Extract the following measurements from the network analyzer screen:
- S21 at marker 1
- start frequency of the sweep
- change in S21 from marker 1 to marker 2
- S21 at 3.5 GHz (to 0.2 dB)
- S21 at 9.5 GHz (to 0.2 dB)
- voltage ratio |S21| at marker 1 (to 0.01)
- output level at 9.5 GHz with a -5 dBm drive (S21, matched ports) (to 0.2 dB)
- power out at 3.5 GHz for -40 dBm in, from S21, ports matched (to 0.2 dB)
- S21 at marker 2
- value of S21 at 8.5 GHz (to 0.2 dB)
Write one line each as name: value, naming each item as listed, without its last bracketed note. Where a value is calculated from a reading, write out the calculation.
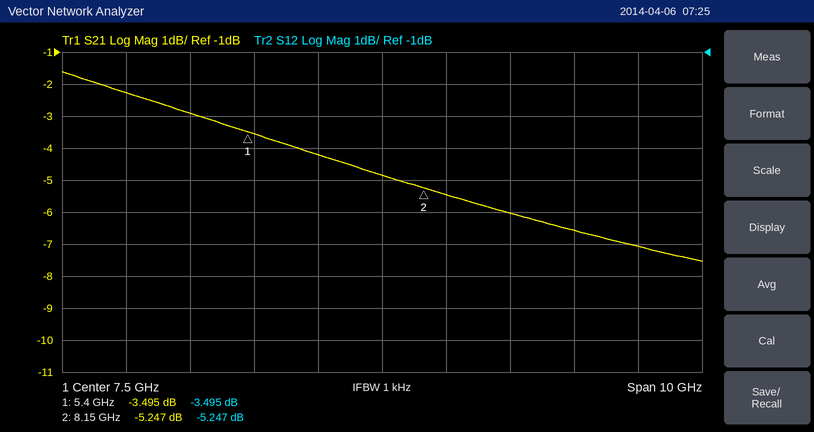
S21 at marker 1: -3.495 dB
start frequency of the sweep: 2.5 GHz
change in S21 from marker 1 to marker 2: -5.247 − (-3.495) = -1.752 dB
S21 at 3.5 GHz: -2.2 dB
S21 at 9.5 GHz: -6.0 dB
voltage ratio |S21| at marker 1: 10^(-3.495/20) ≈ 0.67
output level at 9.5 GHz with a -5 dBm drive (S21, matched ports): -5 dBm + (-6.0 dB) = -11.0 dBm
power out at 3.5 GHz for -40 dBm in, from S21, ports matched: -40 dBm + (-2.2 dB) = -42.2 dBm
S21 at marker 2: -5.247 dB
value of S21 at 8.5 GHz: -5.4 dB
